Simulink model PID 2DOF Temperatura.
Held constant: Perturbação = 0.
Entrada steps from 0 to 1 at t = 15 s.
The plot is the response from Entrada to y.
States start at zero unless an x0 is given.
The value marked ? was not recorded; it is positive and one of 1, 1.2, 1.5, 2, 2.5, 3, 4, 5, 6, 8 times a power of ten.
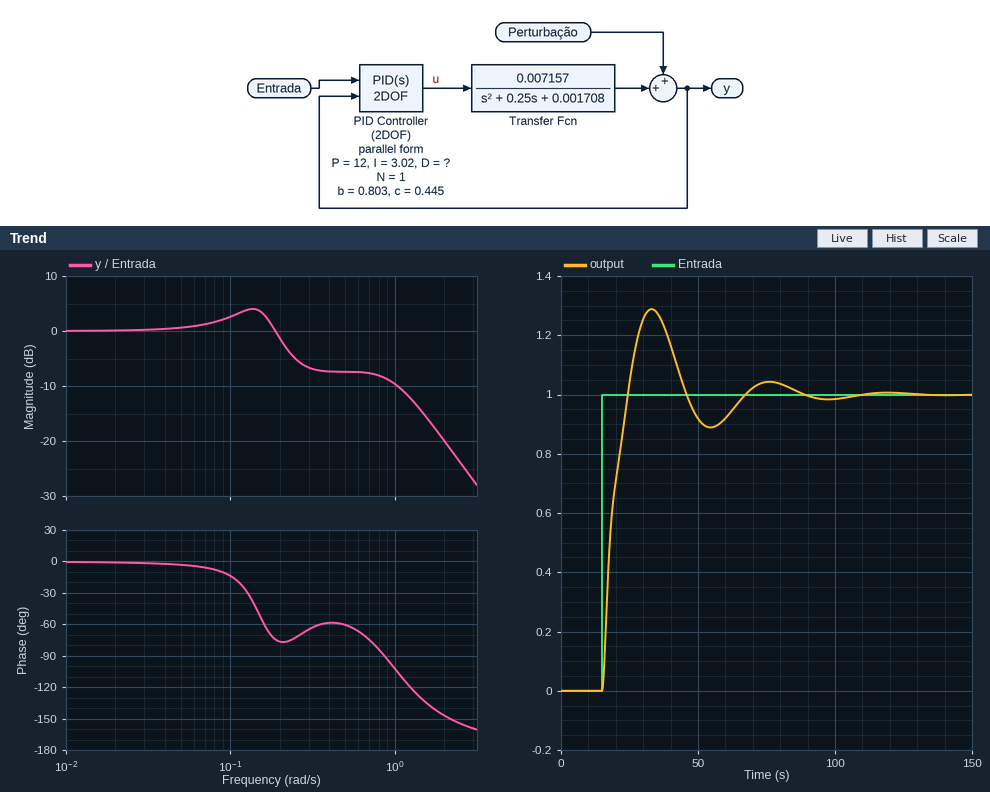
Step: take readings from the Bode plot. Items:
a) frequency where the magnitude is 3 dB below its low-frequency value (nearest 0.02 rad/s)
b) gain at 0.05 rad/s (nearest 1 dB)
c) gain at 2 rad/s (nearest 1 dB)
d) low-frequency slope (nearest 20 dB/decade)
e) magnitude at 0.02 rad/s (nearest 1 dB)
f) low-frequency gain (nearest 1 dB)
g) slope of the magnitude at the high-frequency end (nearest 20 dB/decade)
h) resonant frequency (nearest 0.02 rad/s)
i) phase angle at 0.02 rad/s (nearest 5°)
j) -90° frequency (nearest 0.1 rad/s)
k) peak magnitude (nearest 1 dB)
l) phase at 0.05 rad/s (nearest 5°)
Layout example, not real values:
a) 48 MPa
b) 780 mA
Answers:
a) 0.22 rad/s
b) 1 dB
c) -20 dB
d) 0 dB/decade
e) 0 dB
f) 0 dB
g) -40 dB/decade
h) 0.14 rad/s
i) 0°
j) 0.9 rad/s
k) 4 dB
l) -5°
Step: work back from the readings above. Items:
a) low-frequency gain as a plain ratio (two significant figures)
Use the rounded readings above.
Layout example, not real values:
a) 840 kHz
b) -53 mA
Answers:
a) 1.0
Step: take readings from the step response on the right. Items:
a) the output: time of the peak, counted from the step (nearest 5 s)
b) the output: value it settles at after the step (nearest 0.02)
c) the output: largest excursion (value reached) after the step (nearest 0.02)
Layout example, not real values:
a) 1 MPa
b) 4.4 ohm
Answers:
a) 20 s
b) 1.00
c) 1.28
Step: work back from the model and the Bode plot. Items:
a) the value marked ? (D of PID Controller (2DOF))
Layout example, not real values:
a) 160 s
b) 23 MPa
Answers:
a) 100
